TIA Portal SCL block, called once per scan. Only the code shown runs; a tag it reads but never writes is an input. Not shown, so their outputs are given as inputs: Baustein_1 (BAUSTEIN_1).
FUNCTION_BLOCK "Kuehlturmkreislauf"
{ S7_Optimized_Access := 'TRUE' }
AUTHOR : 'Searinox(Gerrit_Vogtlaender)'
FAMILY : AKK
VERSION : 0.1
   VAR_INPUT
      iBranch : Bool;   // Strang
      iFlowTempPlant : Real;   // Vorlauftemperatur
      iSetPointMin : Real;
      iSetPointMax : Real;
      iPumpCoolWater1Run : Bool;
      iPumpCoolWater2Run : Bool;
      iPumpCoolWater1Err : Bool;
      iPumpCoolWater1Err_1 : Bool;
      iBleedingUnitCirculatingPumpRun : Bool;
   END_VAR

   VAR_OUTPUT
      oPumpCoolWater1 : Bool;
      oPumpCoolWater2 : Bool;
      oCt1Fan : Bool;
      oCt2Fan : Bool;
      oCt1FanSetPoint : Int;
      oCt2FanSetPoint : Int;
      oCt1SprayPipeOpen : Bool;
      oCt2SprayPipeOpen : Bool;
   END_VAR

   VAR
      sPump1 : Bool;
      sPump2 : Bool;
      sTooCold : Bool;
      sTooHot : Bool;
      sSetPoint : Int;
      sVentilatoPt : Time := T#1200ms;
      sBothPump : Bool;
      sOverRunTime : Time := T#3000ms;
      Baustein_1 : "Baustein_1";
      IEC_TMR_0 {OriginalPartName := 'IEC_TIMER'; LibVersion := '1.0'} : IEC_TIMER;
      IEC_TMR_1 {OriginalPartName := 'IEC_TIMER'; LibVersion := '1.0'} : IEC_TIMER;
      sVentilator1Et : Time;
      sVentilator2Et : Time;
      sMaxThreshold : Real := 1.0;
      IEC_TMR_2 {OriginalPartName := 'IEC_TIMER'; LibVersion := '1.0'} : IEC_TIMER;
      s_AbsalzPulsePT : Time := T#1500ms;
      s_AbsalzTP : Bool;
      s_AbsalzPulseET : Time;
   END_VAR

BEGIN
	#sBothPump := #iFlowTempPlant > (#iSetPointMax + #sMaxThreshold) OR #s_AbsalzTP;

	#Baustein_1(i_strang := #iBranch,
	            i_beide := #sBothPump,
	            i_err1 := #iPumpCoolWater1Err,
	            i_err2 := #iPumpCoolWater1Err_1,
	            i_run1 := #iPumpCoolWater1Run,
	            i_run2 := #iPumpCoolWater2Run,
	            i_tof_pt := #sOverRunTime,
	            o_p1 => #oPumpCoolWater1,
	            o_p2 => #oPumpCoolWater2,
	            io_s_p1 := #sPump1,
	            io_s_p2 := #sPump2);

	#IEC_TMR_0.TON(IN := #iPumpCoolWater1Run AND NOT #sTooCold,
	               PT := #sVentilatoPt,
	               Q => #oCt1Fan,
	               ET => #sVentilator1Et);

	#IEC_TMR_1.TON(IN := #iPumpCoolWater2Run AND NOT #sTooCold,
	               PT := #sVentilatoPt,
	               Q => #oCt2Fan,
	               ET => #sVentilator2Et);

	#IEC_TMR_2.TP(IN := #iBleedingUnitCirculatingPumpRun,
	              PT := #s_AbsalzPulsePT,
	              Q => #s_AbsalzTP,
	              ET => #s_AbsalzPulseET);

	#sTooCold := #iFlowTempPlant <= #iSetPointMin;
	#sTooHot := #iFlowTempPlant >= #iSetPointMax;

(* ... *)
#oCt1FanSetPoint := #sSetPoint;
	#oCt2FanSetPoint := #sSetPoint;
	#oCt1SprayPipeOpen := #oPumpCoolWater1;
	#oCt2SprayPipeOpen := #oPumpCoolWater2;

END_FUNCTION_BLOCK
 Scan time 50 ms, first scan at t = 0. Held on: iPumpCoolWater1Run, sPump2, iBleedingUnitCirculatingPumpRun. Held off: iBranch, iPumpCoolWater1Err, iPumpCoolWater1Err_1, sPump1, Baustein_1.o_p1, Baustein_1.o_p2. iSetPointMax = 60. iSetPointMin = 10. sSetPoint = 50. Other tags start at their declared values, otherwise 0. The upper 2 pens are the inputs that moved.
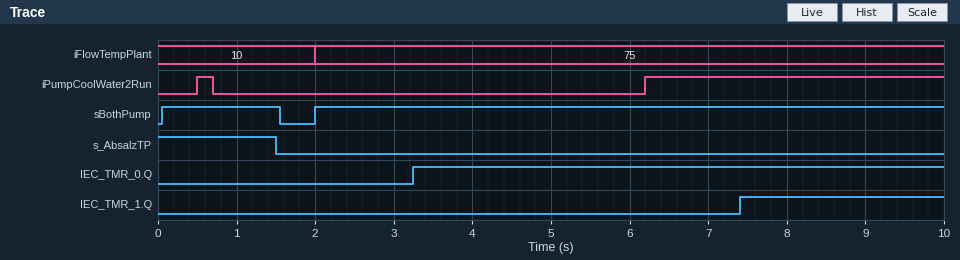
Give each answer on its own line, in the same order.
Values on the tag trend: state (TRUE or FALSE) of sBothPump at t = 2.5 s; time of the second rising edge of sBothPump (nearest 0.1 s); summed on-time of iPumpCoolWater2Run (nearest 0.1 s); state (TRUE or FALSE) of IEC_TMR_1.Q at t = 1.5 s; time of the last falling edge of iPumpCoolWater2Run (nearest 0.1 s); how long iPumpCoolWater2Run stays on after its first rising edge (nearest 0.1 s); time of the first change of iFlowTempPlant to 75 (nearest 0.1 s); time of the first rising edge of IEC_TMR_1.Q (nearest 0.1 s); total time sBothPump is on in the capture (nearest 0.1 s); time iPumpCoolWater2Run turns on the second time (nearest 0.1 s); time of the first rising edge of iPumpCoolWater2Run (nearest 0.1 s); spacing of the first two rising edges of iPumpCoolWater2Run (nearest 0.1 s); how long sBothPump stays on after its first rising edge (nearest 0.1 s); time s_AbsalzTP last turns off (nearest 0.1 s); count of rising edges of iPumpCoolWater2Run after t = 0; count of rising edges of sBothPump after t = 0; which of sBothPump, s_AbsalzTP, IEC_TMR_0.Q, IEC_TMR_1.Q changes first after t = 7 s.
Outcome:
TRUE
2.0 s
4.0 s
FALSE
0.7 s
0.2 s
2.0 s
7.4 s
9.5 s
6.2 s
0.5 s
5.7 s
1.5 s
1.5 s
2
2
IEC_TMR_1.Q
